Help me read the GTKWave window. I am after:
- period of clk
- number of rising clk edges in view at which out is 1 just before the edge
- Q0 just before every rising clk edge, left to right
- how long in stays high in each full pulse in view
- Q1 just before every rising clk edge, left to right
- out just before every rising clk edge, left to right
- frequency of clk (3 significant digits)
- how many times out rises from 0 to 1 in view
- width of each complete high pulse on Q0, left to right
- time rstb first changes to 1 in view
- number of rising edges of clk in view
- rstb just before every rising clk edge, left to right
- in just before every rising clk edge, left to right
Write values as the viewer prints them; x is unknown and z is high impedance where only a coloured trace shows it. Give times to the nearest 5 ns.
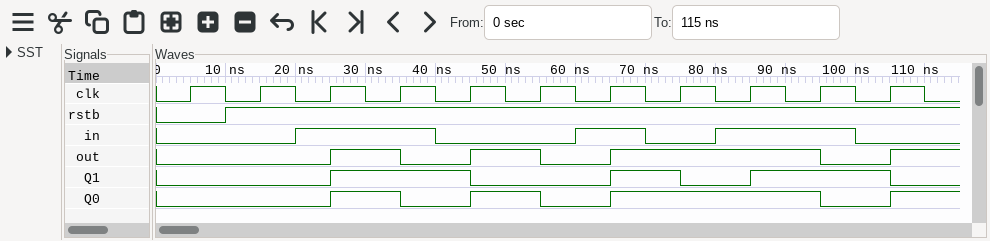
10 ns
5
0 0 0 1 0 1 0 1 1 1 0
20 ns, 10 ns, 20 ns
0 0 0 1 1 0 0 1 0 1 1
0 0 0 1 0 1 0 1 1 1 0
100 MHz
4
10 ns, 10 ns, 30 ns
10 ns
11
0 1 1 1 1 1 1 1 1 1 1
0 0 1 1 0 0 1 0 1 1 0
